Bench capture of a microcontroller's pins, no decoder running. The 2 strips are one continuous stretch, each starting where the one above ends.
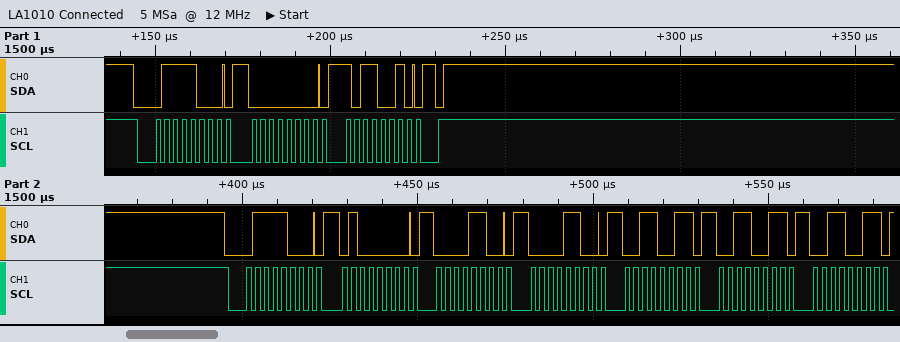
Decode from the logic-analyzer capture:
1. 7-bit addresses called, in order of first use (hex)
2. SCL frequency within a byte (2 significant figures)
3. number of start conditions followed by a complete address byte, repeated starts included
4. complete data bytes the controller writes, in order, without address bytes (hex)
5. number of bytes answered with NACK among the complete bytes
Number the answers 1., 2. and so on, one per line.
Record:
1. 0x3C
2. 400 kHz
3. 2
4. 00 B2 40 0C 0C 33 33 33
5. 0
